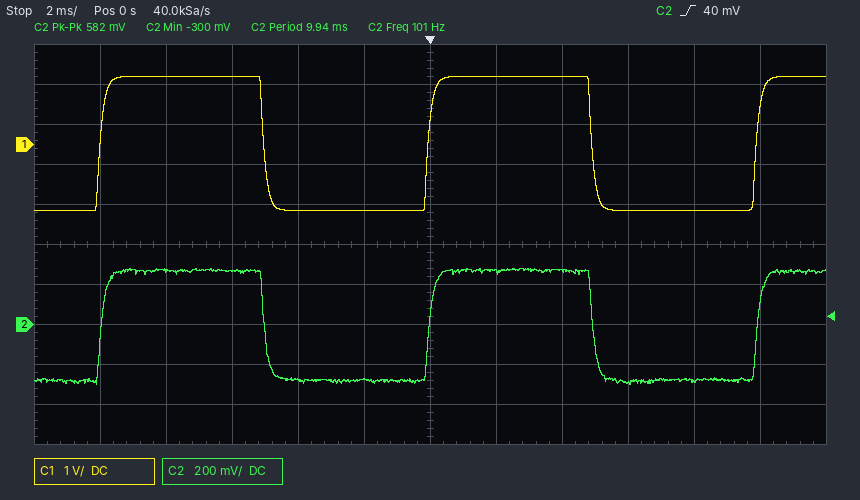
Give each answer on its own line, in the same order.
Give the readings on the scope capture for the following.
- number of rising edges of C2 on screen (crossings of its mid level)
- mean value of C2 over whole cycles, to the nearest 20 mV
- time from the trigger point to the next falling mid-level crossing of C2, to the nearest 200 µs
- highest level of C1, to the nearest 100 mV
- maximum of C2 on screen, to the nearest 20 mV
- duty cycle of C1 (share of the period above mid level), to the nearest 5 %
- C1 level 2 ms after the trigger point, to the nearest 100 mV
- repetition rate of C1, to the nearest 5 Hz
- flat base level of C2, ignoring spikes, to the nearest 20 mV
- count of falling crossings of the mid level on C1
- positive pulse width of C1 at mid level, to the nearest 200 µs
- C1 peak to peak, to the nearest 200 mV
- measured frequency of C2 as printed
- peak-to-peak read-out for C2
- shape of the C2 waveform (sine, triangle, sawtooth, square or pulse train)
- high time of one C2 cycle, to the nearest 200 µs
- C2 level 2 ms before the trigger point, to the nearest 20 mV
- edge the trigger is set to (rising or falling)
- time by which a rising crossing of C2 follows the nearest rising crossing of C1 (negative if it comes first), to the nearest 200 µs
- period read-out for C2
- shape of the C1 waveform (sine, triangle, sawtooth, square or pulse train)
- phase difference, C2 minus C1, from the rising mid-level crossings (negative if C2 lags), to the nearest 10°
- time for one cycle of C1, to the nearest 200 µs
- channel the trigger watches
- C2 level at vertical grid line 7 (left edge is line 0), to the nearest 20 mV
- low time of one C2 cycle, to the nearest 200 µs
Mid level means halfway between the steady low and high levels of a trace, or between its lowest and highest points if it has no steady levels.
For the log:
3
0 mV
5.0 ms
1.7 V
280 mV
50 %
1.7 V
100 Hz
-280 mV
2
5.0 ms
3.4 V
101 Hz
582 mV
square
5.0 ms
-280 mV
rising
0.0 ms
9.94 ms
square
0°
10.0 ms
C2
260 mV
5.0 ms
